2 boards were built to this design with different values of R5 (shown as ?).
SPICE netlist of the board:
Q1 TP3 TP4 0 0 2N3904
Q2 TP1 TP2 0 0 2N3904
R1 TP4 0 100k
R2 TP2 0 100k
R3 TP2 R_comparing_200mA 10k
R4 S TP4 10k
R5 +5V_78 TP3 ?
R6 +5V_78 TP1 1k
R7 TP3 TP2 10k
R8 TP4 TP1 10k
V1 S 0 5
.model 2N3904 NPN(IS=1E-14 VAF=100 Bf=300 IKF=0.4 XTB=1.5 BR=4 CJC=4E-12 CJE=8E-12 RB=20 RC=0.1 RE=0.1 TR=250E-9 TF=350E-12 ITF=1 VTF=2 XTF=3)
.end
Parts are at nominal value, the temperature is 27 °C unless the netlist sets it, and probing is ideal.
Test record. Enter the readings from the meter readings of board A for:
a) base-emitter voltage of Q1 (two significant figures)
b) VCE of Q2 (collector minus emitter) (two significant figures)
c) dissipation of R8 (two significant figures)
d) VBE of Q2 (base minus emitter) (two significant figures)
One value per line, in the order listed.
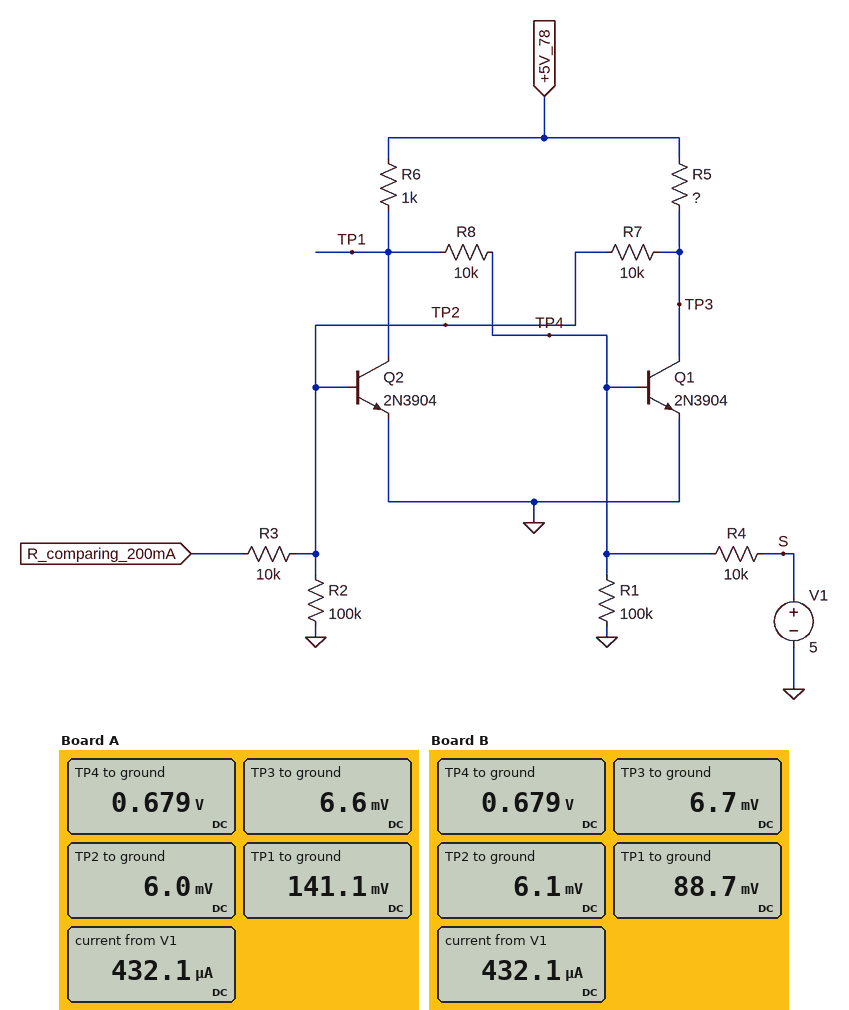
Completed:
680 mV
140 mV
29 µW
6.0 mV
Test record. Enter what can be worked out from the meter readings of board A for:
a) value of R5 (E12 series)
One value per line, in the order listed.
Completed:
1.5 kΩ
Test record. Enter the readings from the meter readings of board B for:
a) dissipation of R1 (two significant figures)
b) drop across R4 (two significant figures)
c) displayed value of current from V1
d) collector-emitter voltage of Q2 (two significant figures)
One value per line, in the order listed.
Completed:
4.6 µW
4.3 V
432.1 µA
89 mV
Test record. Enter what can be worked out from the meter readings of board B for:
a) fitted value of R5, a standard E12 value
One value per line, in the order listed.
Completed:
390 Ω
